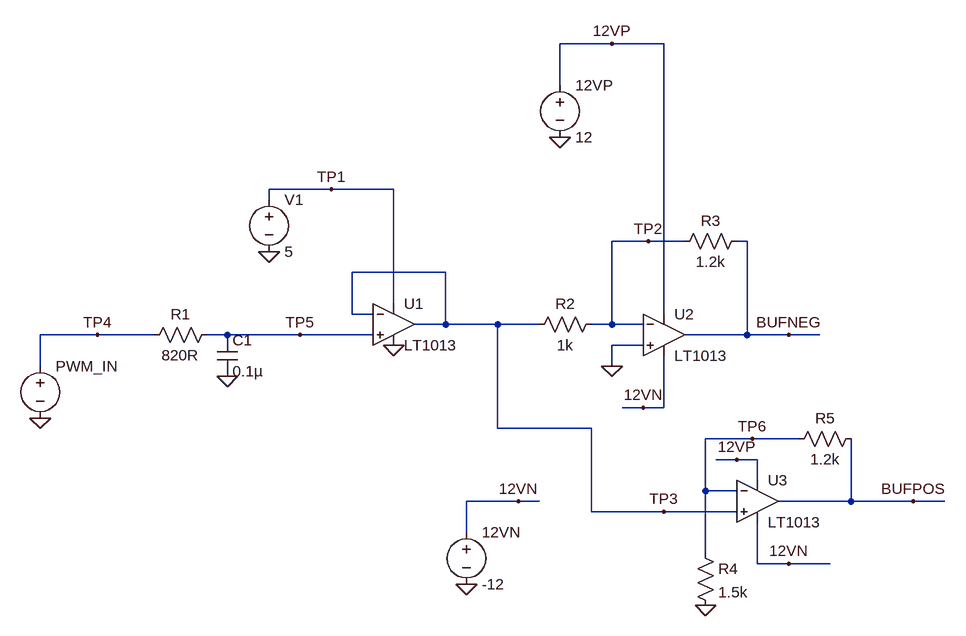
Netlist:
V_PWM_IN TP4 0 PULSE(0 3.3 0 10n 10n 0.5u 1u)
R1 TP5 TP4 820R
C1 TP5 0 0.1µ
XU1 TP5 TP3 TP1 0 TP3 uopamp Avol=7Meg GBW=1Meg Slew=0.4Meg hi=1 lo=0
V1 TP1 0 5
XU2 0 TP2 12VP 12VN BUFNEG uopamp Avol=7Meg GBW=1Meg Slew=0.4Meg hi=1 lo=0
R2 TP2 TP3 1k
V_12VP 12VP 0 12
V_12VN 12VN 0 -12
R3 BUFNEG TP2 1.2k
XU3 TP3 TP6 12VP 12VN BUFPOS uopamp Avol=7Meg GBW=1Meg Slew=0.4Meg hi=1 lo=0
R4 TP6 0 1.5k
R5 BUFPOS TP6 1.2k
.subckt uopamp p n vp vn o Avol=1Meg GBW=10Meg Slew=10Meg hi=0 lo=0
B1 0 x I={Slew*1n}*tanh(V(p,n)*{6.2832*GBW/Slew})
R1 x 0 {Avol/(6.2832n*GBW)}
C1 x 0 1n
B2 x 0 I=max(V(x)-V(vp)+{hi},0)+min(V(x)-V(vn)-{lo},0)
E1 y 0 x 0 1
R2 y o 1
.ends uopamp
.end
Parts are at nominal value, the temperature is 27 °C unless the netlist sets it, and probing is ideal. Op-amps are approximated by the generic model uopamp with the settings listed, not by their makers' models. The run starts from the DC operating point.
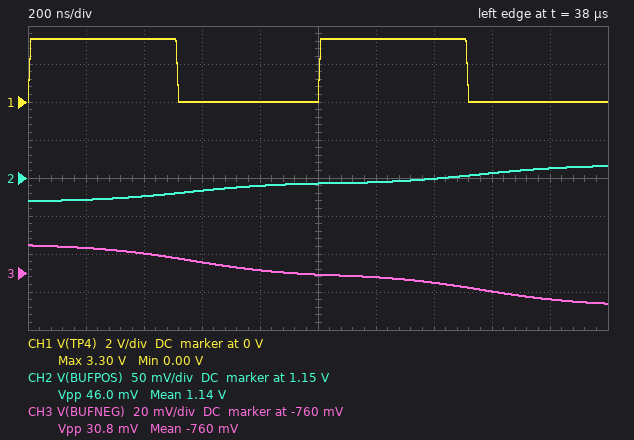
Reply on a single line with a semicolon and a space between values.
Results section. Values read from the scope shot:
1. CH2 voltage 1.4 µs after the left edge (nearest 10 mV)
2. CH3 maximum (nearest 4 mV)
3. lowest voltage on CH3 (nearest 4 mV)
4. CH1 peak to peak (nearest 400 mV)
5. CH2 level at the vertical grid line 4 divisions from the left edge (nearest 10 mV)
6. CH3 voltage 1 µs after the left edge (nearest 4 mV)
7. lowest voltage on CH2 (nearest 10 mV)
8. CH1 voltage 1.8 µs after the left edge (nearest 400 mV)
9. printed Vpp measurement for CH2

1.15 V; -744 mV; -776 mV; 3.2 V; 1.14 V; -760 mV; 1.12 V; 0 V; 46.0 mV
